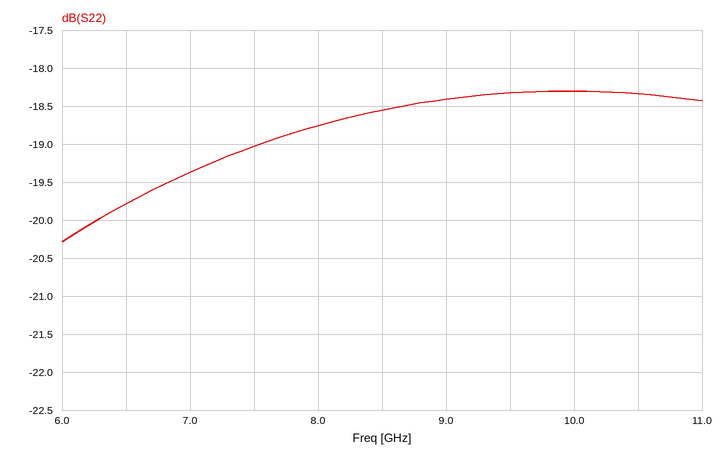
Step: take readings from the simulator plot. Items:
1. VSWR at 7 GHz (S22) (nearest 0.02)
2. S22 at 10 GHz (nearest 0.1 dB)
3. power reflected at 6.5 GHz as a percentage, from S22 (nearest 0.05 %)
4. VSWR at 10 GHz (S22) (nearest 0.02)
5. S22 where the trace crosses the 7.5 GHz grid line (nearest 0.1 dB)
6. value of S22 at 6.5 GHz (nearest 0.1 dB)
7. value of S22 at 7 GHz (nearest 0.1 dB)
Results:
1.24
-18.3 dB
1.05 %
1.28
-19.0 dB
-19.8 dB
-19.4 dB
